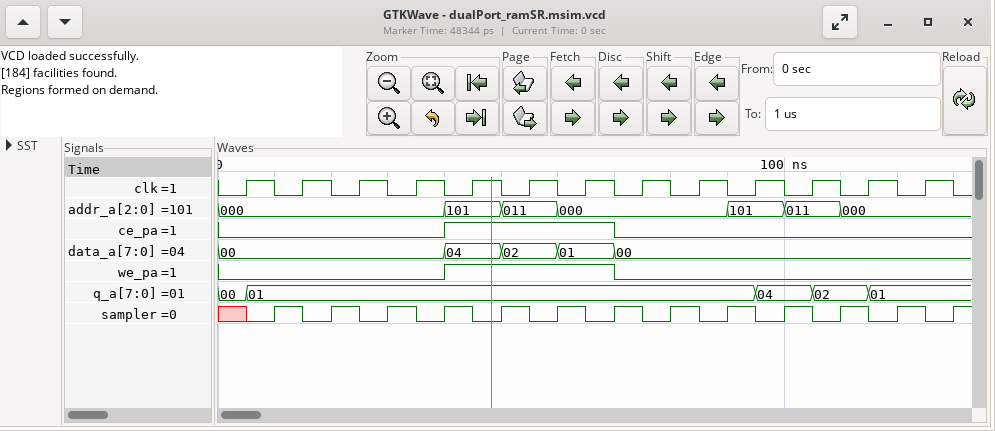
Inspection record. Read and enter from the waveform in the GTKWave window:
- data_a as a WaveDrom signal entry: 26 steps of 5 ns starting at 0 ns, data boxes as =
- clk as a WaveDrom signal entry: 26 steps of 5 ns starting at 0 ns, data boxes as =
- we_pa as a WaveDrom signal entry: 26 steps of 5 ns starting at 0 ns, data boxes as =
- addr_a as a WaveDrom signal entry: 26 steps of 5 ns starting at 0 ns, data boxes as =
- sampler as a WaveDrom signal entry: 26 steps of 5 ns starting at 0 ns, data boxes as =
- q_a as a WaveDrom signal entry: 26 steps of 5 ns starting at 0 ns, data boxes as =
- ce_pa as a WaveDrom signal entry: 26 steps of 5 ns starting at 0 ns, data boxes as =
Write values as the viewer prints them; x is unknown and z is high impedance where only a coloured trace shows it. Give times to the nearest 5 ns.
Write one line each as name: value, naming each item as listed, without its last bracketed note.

data_a as a WaveDrom signal entry: 26 steps of 5 ns starting at 0 ns, data boxes as =: {name: 'data_a', wave: '=.......=.=.=.=...........', data: '00 04 02 01 00'}
clk as a WaveDrom signal entry: 26 steps of 5 ns starting at 0 ns, data boxes as =: {name: 'clk', wave: '01010101010101010101010101'}
we_pa as a WaveDrom signal entry: 26 steps of 5 ns starting at 0 ns, data boxes as =: {name: 'we_pa', wave: '0.......1.....0...........'}
addr_a as a WaveDrom signal entry: 26 steps of 5 ns starting at 0 ns, data boxes as =: {name: 'addr_a', wave: '=.......=.=.=.....=.=.=...', data: '000 101 011 000 101 011 000'}
sampler as a WaveDrom signal entry: 26 steps of 5 ns starting at 0 ns, data boxes as =: {name: 'sampler', wave: 'x0101010101010101010101010'}
q_a as a WaveDrom signal entry: 26 steps of 5 ns starting at 0 ns, data boxes as =: {name: 'q_a', wave: '==.................=.=.=..', data: '00 01 04 02 01'}
ce_pa as a WaveDrom signal entry: 26 steps of 5 ns starting at 0 ns, data boxes as =: {name: 'ce_pa', wave: '0.......1.....0...........'}
